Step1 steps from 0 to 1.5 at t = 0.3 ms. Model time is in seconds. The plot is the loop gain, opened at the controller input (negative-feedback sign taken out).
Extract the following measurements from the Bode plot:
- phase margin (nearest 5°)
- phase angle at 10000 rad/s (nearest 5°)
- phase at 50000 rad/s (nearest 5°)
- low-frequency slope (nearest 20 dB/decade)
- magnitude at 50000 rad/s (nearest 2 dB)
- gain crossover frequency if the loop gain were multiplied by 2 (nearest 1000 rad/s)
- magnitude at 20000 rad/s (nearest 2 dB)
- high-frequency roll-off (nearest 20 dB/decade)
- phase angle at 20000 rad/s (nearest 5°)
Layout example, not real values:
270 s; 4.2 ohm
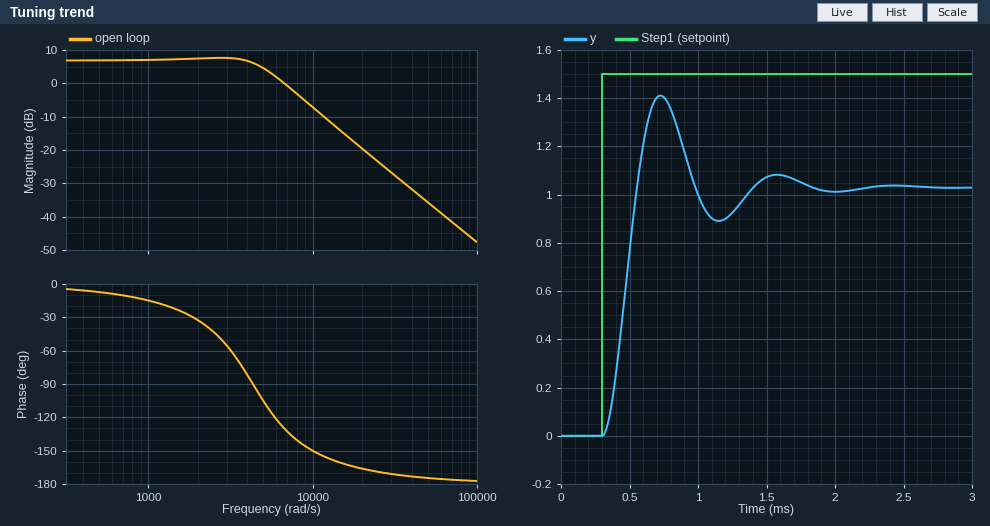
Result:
50°; -150°; -175°; 0 dB/decade; -36 dB; 9000 rad/s; -20 dB; -40 dB/decade; -165°
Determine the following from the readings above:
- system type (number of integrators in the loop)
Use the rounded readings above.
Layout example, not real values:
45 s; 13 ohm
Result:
0
